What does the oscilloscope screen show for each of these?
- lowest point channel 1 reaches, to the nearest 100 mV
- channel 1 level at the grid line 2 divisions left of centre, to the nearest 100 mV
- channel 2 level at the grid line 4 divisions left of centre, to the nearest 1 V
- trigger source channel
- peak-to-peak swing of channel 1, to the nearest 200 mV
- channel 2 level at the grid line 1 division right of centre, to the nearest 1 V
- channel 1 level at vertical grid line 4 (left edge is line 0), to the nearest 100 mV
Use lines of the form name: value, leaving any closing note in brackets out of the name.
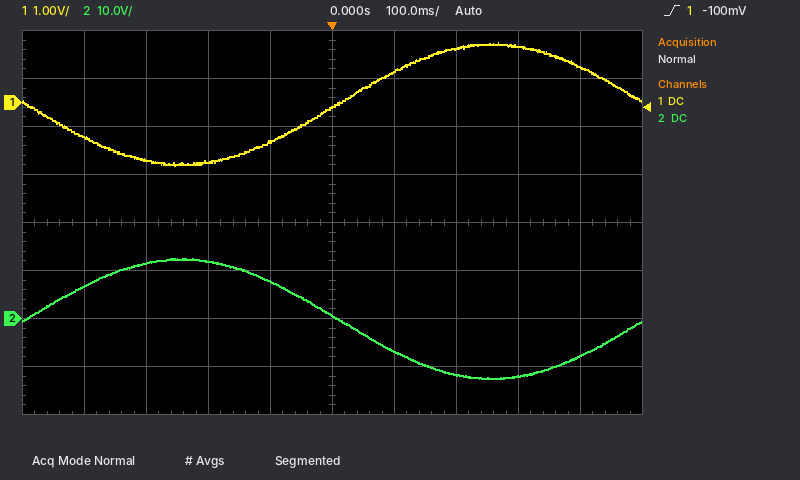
lowest point channel 1 reaches, to the nearest 100 mV: -1.3 V
channel 1 level at the grid line 2 divisions left of centre, to the nearest 100 mV: -1.2 V
channel 2 level at the grid line 4 divisions left of centre, to the nearest 1 V: 7 V
trigger source channel: channel 1
peak-to-peak swing of channel 1, to the nearest 200 mV: 2.6 V
channel 2 level at the grid line 1 division right of centre, to the nearest 1 V: -7 V
channel 1 level at vertical grid line 4 (left edge is line 0), to the nearest 100 mV: -800 mV
